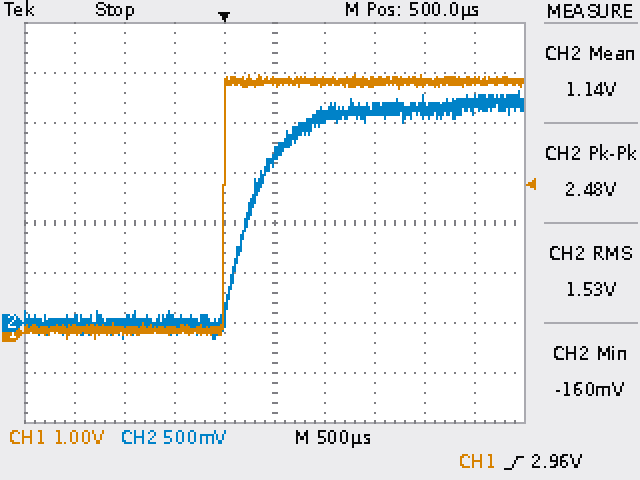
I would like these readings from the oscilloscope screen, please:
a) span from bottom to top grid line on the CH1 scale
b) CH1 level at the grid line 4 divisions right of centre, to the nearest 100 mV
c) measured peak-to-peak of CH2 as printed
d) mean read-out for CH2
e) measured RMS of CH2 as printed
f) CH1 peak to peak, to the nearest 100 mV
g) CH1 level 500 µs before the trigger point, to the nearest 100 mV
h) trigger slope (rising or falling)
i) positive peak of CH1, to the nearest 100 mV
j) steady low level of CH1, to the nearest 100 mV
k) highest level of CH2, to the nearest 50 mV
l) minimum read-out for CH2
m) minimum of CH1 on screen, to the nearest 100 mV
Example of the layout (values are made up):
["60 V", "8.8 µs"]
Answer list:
["8 V", "5.0 V", "2.48 V", "1.14 V", "1.53 V", "5.3 V", "100 mV", "rising", "5.2 V", "100 mV", "2.30 V", "-160 mV", "-100 mV"]
